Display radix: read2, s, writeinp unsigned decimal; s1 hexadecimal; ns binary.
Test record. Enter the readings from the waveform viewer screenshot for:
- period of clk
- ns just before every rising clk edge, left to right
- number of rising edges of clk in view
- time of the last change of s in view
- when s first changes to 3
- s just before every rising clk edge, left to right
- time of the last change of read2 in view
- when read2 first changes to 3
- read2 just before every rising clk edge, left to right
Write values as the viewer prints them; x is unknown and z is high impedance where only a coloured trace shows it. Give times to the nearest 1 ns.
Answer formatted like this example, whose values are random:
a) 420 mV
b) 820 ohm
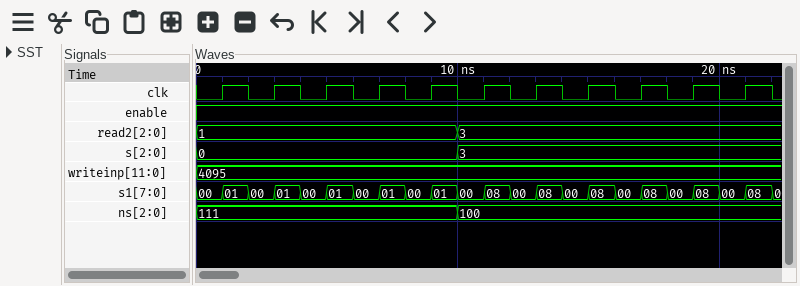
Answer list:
a) 2 ns
b) 111, 111, 111, 111, 111, 100, 100, 100, 100, 100, 100
c) 11
d) 10 ns
e) 10 ns
f) 0, 0, 0, 0, 0, 3, 3, 3, 3, 3, 3
g) 10 ns
h) 10 ns
i) 1, 1, 1, 1, 1, 3, 3, 3, 3, 3, 3
